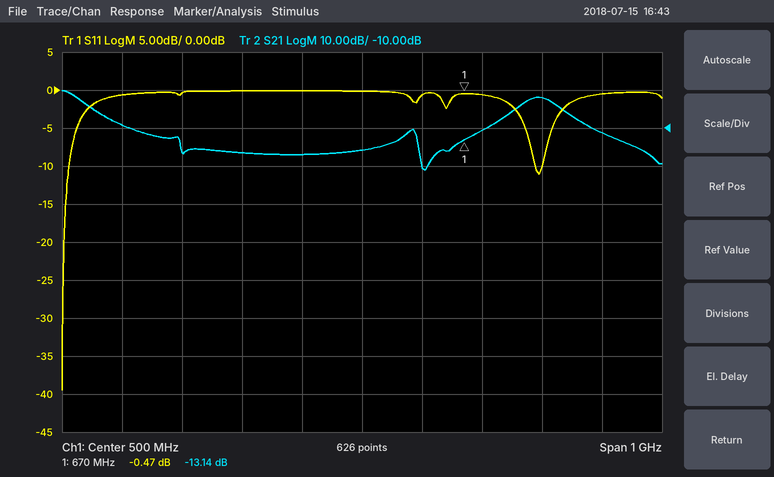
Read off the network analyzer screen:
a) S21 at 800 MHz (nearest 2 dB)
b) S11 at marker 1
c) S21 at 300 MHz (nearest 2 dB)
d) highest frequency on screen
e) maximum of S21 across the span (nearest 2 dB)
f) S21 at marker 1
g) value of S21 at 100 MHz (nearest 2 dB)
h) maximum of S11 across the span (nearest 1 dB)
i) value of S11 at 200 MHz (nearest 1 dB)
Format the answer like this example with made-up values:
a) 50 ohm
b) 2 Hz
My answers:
a) -2 dB
b) -0.47 dB
c) -16 dB
d) 1 GHz
e) 0 dB
f) -13.14 dB
g) -10 dB
h) 0 dB
i) 0 dB
